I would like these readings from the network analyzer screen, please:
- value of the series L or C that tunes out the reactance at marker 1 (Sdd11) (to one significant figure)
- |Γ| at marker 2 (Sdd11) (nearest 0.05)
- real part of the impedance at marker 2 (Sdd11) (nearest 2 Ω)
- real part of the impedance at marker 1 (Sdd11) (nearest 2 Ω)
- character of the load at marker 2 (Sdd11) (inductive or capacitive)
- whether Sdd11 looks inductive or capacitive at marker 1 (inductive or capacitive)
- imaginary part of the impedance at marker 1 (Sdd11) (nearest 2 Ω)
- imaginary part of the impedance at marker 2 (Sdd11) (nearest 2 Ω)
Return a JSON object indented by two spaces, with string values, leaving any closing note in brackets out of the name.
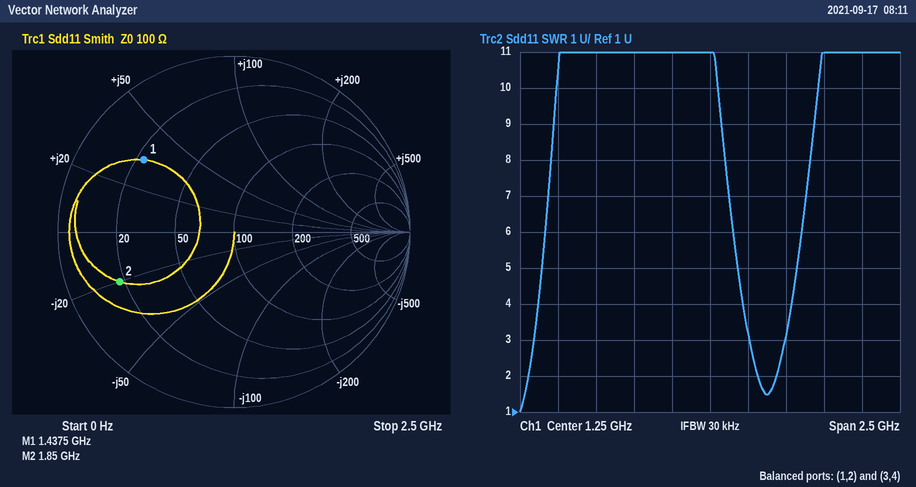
{
  "value of the series L or C that tunes out the reactance at marker 1 (Sdd11)": "3 pF",
  "|Γ| at marker 2 (Sdd11)": "0.70",
  "real part of the impedance at marker 2 (Sdd11)": "18 Ω",
  "real part of the impedance at marker 1 (Sdd11)": "24 Ω",
  "character of the load at marker 2 (Sdd11)": "capacitive",
  "whether Sdd11 looks inductive or capacitive at marker 1": "inductive",
  "imaginary part of the impedance at marker 1 (Sdd11)": "+34 Ω",
  "imaginary part of the impedance at marker 2 (Sdd11)": "-20 Ω"
}
